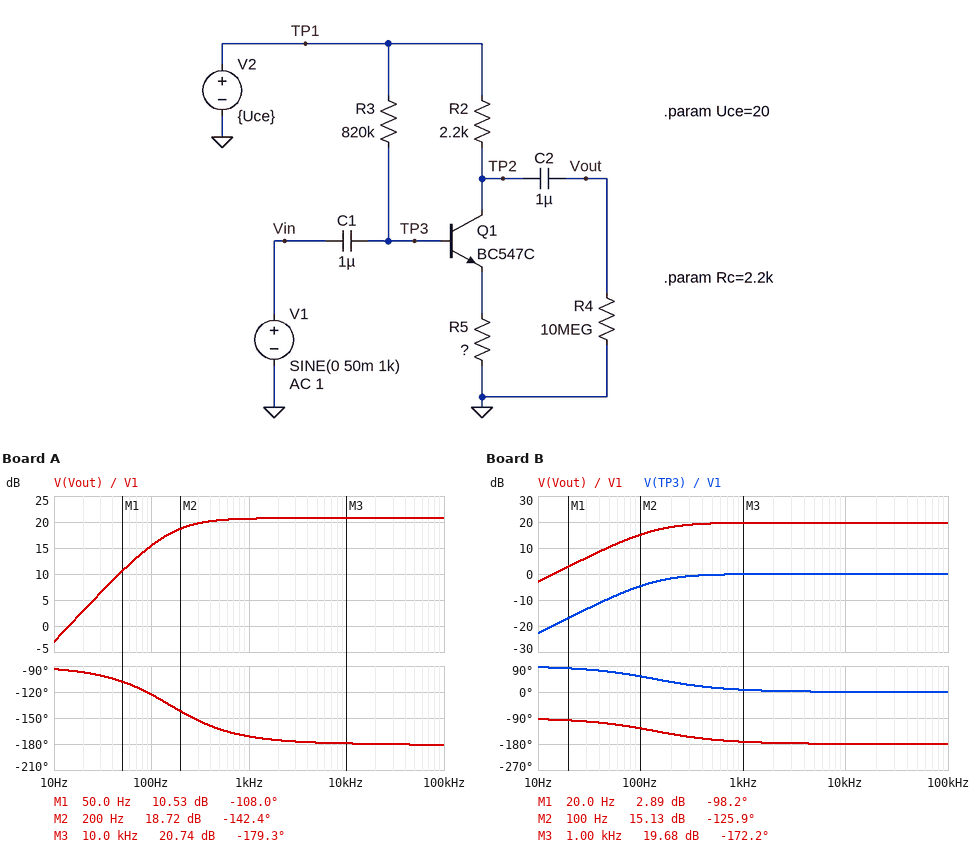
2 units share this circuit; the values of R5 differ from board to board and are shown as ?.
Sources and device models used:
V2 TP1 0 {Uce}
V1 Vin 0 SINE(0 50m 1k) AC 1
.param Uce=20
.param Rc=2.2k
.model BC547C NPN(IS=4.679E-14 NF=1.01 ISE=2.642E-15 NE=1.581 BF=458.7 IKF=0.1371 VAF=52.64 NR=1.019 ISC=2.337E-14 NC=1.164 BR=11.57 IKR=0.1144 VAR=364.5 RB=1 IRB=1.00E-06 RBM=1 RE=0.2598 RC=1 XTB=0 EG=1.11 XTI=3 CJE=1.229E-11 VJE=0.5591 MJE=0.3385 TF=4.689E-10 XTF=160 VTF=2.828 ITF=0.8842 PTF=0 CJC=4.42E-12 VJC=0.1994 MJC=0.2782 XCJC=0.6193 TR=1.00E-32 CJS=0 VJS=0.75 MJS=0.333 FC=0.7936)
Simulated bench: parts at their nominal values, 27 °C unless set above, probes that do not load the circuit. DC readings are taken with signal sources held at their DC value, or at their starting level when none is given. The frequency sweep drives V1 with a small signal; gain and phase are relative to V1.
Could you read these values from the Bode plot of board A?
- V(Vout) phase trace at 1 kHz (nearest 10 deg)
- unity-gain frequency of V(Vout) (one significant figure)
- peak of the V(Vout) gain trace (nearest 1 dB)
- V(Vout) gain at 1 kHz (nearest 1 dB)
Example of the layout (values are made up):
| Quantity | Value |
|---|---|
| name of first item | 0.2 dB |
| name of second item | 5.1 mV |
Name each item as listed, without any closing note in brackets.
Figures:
| Quantity | Value |
|---|---|
| V(Vout) phase trace at 1 kHz | -170 deg |
| unity-gain frequency of V(Vout) | 10 Hz |
| peak of the V(Vout) gain trace | 21 dB |
| V(Vout) gain at 1 kHz | 21 dB |
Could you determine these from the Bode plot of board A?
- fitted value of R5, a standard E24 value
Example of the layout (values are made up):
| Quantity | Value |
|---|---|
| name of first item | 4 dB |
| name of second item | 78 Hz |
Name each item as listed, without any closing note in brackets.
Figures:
| Quantity | Value |
|---|---|
| fitted value of R5, a standard E24 value | 160 Ω |
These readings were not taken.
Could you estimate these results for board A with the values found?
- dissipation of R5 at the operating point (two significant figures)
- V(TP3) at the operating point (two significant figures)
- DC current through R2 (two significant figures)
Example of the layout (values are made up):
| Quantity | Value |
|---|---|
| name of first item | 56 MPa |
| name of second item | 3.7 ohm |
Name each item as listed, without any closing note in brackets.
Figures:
| Quantity | Value |
|---|---|
| dissipation of R5 at the operating point | 11 mW |
| V(TP3) at the operating point | 2.0 V |
| DC current through R2 | 8.4 mA |
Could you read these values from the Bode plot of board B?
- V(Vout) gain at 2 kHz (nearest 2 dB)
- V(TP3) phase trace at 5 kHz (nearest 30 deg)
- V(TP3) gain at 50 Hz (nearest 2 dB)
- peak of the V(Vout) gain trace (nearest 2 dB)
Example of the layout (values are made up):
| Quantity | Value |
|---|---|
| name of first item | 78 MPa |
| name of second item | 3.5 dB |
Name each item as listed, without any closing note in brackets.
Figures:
| Quantity | Value |
|---|---|
| V(Vout) gain at 2 kHz | 20 dB |
| V(TP3) phase trace at 5 kHz | 0 deg |
| V(TP3) gain at 50 Hz | -10 dB |
| peak of the V(Vout) gain trace | 20 dB |
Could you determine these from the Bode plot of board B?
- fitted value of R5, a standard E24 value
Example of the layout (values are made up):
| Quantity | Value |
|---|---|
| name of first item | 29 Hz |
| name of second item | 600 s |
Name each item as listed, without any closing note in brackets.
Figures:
| Quantity | Value |
|---|---|
| fitted value of R5, a standard E24 value | 180 Ω |
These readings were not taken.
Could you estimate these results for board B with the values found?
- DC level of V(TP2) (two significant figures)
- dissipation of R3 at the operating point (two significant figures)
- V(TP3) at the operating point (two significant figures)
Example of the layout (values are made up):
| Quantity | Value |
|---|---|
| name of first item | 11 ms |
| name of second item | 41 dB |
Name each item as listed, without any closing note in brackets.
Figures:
| Quantity | Value |
|---|---|
| DC level of V(TP2) | 1.7 V |
| dissipation of R3 at the operating point | 390 µW |
| V(TP3) at the operating point | 2.2 V |
